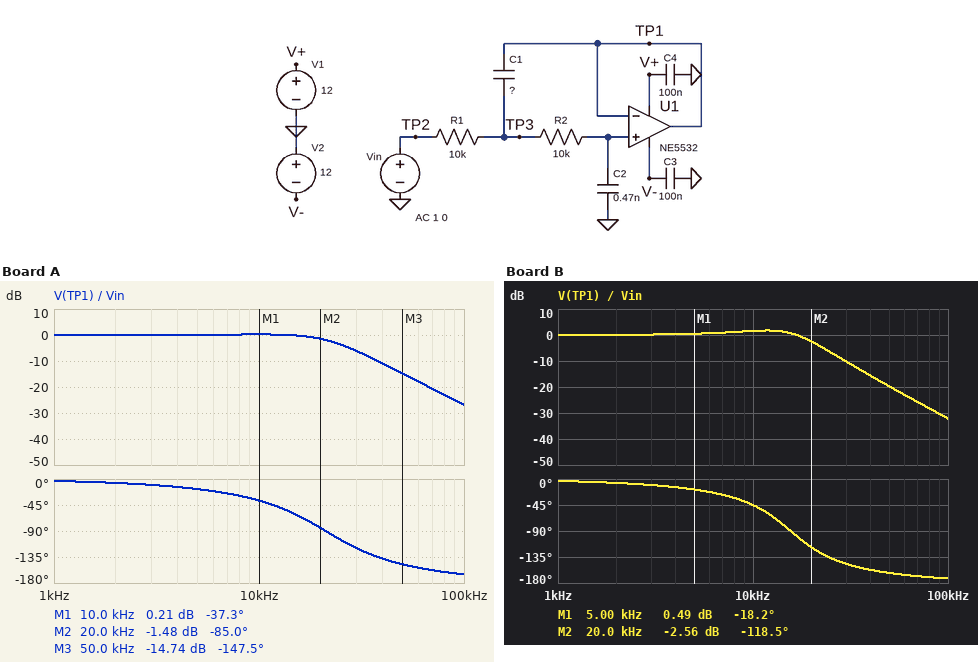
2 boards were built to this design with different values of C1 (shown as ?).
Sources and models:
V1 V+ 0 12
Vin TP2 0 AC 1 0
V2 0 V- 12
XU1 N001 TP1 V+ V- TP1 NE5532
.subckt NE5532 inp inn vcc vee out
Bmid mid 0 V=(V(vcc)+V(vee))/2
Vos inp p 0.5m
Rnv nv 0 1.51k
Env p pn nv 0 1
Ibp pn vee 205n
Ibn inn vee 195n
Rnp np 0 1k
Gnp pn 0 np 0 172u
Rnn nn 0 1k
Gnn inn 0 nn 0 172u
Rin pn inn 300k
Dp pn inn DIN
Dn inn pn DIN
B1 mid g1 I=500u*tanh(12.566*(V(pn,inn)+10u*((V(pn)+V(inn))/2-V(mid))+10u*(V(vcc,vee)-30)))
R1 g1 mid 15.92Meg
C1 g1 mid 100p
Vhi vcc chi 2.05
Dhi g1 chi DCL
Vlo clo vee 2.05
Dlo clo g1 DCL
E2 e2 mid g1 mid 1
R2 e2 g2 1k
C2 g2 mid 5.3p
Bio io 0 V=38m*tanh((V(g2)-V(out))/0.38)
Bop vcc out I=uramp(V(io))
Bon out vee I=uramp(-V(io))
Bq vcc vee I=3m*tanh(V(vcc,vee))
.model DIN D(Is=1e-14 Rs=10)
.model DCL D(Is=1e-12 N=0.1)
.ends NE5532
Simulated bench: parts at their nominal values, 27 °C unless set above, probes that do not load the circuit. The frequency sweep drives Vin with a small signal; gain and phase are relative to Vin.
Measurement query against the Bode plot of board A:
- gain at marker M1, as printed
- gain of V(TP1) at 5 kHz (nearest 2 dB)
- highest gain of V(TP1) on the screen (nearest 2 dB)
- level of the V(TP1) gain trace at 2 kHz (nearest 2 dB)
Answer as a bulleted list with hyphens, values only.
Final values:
- 0.21 dB
- 0 dB
- 0 dB
- 0 dB
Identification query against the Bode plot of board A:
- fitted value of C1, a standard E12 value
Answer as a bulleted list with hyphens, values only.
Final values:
- 1.2 nF
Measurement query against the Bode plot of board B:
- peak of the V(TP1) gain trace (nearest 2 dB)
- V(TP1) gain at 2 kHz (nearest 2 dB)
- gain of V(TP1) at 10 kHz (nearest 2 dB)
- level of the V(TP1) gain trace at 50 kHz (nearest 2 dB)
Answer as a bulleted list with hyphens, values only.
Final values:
- 2 dB
- 0 dB
- 2 dB
- -20 dB
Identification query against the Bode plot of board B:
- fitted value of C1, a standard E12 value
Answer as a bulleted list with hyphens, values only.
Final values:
- 2.2 nF
